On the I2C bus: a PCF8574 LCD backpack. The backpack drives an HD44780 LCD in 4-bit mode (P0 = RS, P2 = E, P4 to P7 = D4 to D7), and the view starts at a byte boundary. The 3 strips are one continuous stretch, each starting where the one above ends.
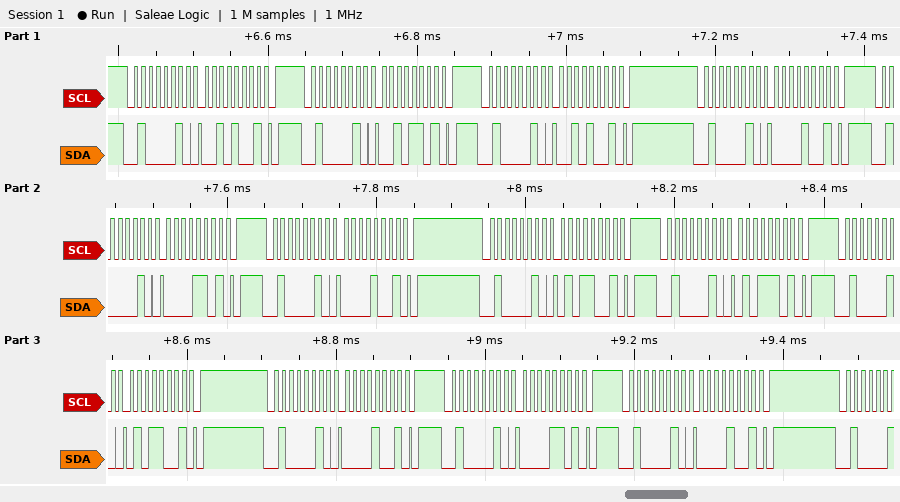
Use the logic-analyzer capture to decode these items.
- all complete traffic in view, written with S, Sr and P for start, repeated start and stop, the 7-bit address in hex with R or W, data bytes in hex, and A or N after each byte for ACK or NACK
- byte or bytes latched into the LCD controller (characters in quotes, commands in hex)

S 21W A 29 A P S 21W A 2D A P S 21W A 29 A P S 21W A 09 A P S 21W A 0D A P S 21W A 09 A P S 21W A 59 A P S 21W A 5D A P S 21W A 59 A P S 21W A 09 A P S 21W A 0D A P S 21W A 09 A P
' ' 'P'
